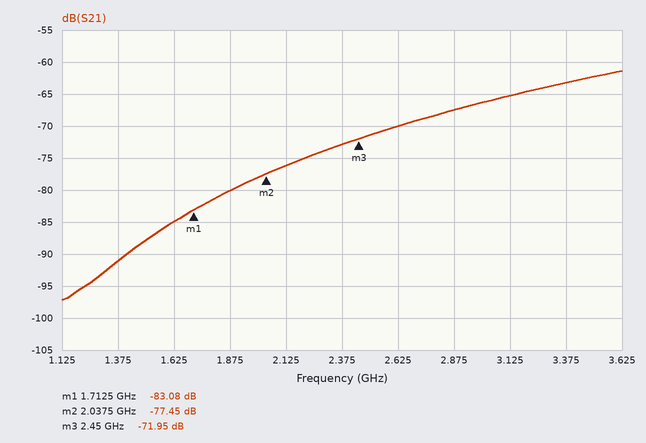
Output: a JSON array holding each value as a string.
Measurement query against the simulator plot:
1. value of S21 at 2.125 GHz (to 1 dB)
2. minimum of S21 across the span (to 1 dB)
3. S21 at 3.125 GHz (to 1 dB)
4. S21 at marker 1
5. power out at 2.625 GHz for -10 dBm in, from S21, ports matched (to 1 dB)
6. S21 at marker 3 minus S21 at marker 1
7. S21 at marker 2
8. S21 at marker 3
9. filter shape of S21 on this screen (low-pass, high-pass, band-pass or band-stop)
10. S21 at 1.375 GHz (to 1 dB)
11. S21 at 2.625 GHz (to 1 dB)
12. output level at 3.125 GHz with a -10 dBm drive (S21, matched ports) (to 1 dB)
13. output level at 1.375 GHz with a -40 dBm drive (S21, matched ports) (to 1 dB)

["-76 dB", "-97 dB", "-65 dB", "-83.08 dB", "-80 dBm", "11.13 dB", "-77.45 dB", "-71.95 dB", "high-pass", "-91 dB", "-70 dB", "-75 dBm", "-131 dBm"]
